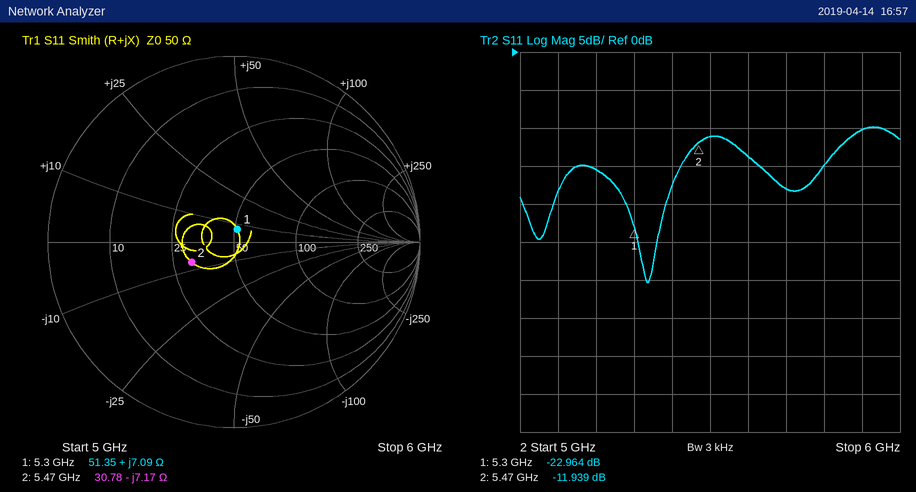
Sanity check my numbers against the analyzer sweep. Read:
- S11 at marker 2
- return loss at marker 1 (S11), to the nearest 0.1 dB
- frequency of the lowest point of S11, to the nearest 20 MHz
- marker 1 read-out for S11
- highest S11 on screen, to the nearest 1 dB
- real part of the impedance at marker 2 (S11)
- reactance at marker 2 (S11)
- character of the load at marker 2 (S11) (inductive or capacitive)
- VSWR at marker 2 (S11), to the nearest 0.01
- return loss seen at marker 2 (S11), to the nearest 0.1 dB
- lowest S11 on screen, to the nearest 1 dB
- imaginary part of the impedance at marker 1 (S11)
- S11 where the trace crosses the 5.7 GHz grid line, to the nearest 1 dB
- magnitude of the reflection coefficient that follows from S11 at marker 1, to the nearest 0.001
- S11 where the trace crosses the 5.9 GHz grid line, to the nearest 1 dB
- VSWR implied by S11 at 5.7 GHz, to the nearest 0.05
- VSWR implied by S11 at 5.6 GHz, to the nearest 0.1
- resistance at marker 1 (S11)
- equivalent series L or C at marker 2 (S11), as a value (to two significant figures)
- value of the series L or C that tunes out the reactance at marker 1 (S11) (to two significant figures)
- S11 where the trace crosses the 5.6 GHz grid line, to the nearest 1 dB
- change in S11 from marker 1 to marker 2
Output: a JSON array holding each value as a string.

["-11.939 dB", "23.0 dB", "5.34 GHz", "-22.964 dB", "-10 dB", "30.78 Ω", "-7.17 Ω", "capacitive", "1.68", "11.9 dB", "-30 dB", "+7.09 Ω", "-18 dB", "0.071", "-10 dB", "1.30", "1.5", "51.35 Ω", "4.1 pF", "4.2 pF", "-14 dB", "11.025 dB"]
